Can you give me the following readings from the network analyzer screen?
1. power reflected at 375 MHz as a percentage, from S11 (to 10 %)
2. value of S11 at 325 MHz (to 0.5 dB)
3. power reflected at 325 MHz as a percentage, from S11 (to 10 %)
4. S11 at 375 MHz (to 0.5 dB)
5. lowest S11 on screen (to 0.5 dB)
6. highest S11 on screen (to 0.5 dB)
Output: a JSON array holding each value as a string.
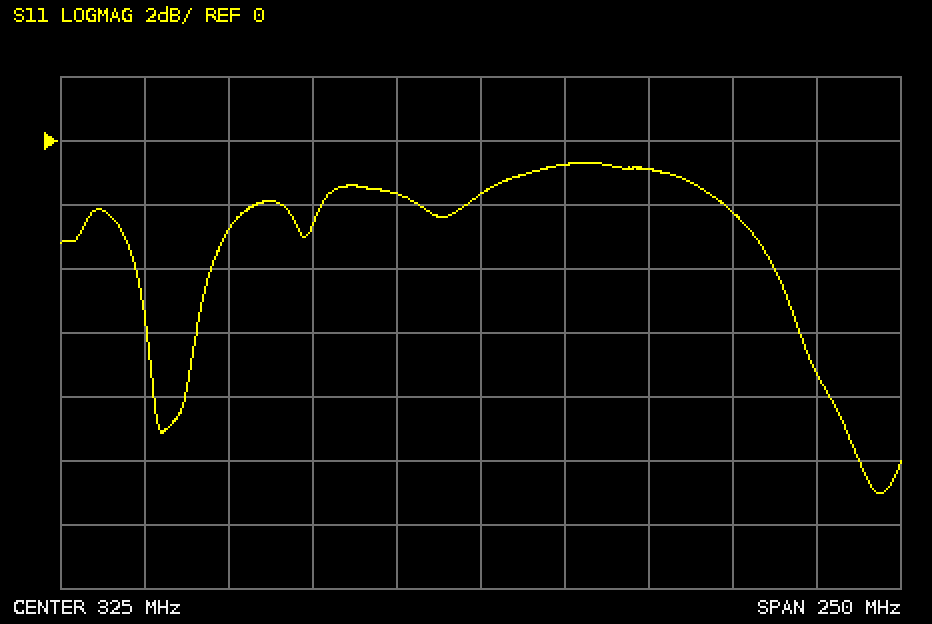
["80 %", "-1.5 dB", "70 %", "-1.0 dB", "-11.0 dB", "-0.5 dB"]
